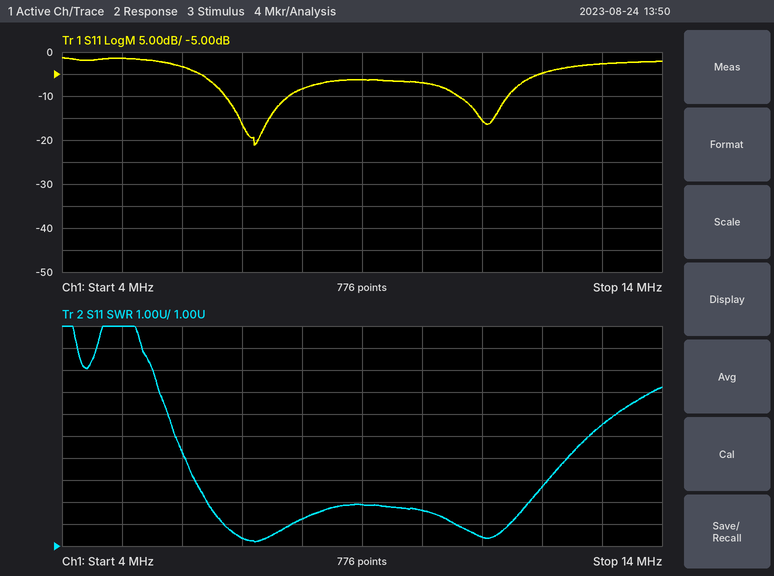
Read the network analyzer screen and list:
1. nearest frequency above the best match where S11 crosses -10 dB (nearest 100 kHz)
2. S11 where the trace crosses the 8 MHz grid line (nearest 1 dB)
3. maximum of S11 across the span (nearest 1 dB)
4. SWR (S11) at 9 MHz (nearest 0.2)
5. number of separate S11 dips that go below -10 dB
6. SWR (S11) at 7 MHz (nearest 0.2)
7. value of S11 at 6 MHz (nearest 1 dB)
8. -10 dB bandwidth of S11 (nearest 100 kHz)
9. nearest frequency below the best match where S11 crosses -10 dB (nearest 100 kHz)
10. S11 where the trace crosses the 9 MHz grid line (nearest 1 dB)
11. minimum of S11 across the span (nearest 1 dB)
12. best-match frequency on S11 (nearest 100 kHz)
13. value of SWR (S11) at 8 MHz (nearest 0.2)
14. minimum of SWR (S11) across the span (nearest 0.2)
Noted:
7.8 MHz
-8 dB
-1 dB
2.8
2
1.4
-3 dB
1.1 MHz
6.7 MHz
-6 dB
-21 dB
7.2 MHz
2.2
1.2
